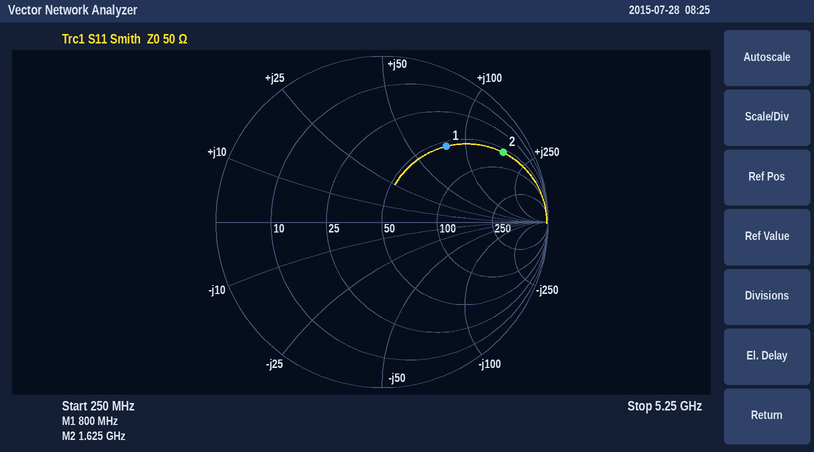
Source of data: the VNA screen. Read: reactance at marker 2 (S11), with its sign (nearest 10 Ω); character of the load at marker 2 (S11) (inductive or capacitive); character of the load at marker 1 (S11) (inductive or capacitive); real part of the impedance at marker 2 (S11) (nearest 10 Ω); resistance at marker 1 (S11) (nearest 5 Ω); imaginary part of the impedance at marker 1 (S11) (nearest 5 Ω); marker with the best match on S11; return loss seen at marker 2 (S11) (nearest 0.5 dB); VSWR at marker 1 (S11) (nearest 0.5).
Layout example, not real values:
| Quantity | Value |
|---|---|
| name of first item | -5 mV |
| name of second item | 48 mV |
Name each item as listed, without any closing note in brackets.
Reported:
| Quantity | Value |
|---|---|
| reactance at marker 2 (S11), with its sign | +170 Ω |
| character of the load at marker 2 (S11) | inductive |
| character of the load at marker 1 (S11) | inductive |
| real part of the impedance at marker 2 (S11) | 60 Ω |
| resistance at marker 1 (S11) | 55 Ω |
| imaginary part of the impedance at marker 1 (S11) | +80 Ω |
| marker with the best match on S11 | marker 1 |
| return loss seen at marker 2 (S11) | 1.5 dB |
| VSWR at marker 1 (S11) | 4.0 |
